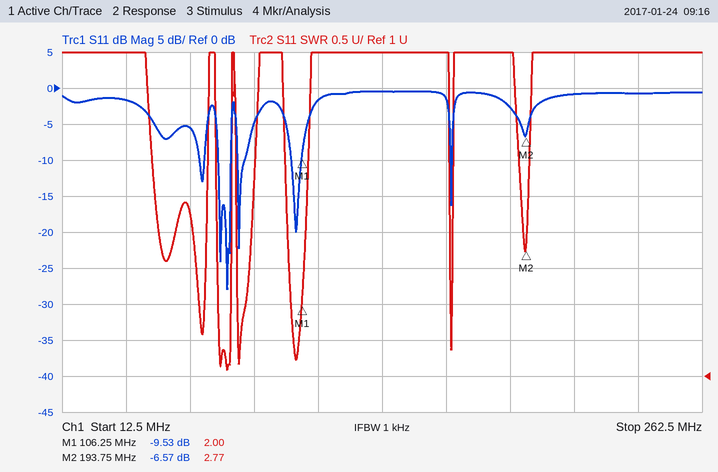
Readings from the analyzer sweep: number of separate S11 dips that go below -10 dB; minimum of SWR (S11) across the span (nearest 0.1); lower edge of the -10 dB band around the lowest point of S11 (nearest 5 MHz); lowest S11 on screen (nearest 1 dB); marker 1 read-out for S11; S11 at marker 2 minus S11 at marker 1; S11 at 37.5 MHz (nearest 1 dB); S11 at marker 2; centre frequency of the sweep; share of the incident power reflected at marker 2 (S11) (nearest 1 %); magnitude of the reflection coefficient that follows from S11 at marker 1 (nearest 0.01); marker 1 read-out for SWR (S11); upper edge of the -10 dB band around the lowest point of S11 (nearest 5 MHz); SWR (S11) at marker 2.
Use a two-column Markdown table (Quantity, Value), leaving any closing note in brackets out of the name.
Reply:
| Quantity | Value |
|---|---|
| number of separate S11 dips that go below -10 dB | 6 |
| minimum of SWR (S11) across the span | 1.1 |
| lower edge of the -10 dB band around the lowest point of S11 | 75 MHz |
| lowest S11 on screen | -28 dB |
| marker 1 read-out for S11 | -9.53 dB |
| S11 at marker 2 minus S11 at marker 1 | 2.96 dB |
| S11 at 37.5 MHz | -2 dB |
| S11 at marker 2 | -6.57 dB |
| centre frequency of the sweep | 137.5 MHz |
| share of the incident power reflected at marker 2 (S11) | 22 % |
| magnitude of the reflection coefficient that follows from S11 at marker 1 | 0.33 |
| marker 1 read-out for SWR | 2.00 |
| upper edge of the -10 dB band around the lowest point of S11 | 80 MHz |
| SWR (S11) at marker 2 | 2.77 |
